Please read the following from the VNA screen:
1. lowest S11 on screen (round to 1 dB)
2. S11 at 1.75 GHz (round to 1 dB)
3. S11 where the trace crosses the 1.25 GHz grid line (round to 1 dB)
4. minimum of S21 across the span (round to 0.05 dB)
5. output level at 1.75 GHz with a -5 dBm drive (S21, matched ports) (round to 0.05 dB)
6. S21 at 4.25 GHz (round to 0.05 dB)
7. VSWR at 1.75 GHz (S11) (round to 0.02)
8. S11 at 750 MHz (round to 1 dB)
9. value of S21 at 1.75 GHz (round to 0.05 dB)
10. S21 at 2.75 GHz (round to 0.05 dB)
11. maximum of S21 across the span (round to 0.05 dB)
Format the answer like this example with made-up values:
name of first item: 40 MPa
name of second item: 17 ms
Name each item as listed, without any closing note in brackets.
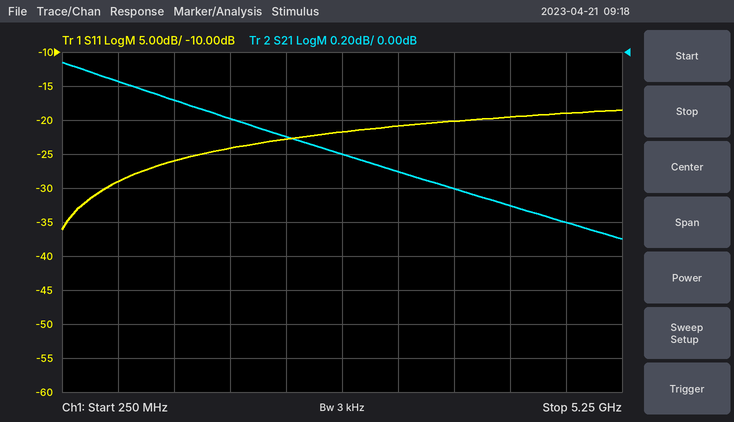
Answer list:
lowest S11 on screen: -36 dB
S11 at 1.75 GHz: -24 dB
S11 where the trace crosses the 1.25 GHz grid line: -26 dB
minimum of S21 across the span: -1.10 dB
output level at 1.75 GHz with a -5 dBm drive (S21, matched ports): -5.40 dBm
S21 at 4.25 GHz: -0.90 dB
VSWR at 1.75 GHz (S11): 1.14
S11 at 750 MHz: -29 dB
value of S21 at 1.75 GHz: -0.40 dB
S21 at 2.75 GHz: -0.60 dB
maximum of S21 across the span: -0.05 dB
